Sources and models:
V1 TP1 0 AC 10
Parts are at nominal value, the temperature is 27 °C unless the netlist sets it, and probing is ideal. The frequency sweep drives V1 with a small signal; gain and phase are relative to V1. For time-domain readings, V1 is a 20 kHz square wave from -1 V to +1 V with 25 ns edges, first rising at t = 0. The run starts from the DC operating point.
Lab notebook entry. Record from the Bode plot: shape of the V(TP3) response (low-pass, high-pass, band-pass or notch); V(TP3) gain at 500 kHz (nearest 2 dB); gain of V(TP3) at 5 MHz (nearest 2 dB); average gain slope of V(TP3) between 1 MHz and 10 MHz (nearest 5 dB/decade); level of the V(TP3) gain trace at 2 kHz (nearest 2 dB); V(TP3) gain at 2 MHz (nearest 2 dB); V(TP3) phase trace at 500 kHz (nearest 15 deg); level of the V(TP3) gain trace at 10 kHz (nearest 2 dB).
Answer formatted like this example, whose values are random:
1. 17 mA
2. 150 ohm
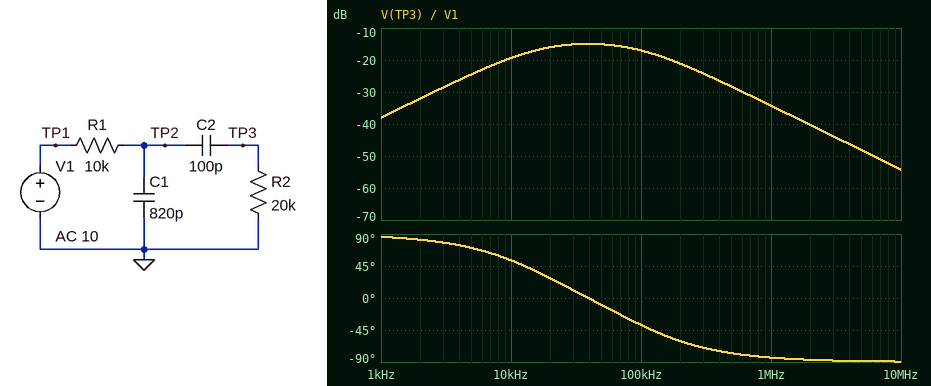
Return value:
1. band-pass
2. -28 dB
3. -48 dB
4. -20 dB/decade
5. -32 dB
6. -40 dB
7. -75 deg
8. -20 dB
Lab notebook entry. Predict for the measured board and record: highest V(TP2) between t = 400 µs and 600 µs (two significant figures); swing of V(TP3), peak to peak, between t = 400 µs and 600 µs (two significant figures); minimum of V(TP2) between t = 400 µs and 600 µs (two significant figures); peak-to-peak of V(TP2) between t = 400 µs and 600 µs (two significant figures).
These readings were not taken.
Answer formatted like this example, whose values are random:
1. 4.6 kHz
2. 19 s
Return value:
1. 870 mV
2. 530 mV
3. -870 mV
4. 1.7 V
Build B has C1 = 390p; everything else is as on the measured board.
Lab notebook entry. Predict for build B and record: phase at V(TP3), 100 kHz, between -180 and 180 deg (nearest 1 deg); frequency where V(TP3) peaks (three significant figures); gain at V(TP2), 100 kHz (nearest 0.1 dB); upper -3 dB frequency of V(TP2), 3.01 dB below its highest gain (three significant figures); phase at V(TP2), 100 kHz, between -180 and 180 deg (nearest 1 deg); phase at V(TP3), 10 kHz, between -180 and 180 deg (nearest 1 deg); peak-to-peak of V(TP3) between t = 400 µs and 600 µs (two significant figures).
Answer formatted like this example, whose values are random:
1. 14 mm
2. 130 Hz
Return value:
1. -26 deg
2. 57.0 kHz
3. -9.5 dB
4. 31.0 kHz
5. -64 deg
6. 66 deg
7. 900 mV
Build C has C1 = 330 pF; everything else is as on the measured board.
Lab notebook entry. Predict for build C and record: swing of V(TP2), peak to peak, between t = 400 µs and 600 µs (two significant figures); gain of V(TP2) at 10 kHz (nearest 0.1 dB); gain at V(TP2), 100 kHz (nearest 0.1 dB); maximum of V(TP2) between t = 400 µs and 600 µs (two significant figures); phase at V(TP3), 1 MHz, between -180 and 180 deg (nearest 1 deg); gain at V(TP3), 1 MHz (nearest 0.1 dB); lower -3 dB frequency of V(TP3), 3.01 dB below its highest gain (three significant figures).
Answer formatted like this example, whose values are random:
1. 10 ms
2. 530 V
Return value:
1. 2.0 V
2. -0.4 dB
3. -8.5 dB
4. 990 mV
5. -81 deg
6. -26.4 dB
7. 22.1 kHz
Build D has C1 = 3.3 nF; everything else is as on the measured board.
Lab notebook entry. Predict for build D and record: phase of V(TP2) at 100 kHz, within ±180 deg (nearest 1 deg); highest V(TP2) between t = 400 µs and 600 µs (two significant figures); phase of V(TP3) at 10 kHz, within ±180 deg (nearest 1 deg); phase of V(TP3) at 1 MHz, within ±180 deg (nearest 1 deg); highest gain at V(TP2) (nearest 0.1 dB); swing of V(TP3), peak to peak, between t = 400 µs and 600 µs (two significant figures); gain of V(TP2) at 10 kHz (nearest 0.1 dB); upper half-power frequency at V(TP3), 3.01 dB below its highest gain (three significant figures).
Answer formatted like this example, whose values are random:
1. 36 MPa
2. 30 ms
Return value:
1. -86 deg
2. 350 mV
3. 18 deg
4. -85 deg
5. 0 dB
6. 130 mV
7. -7.5 dB
8. 91.0 kHz
